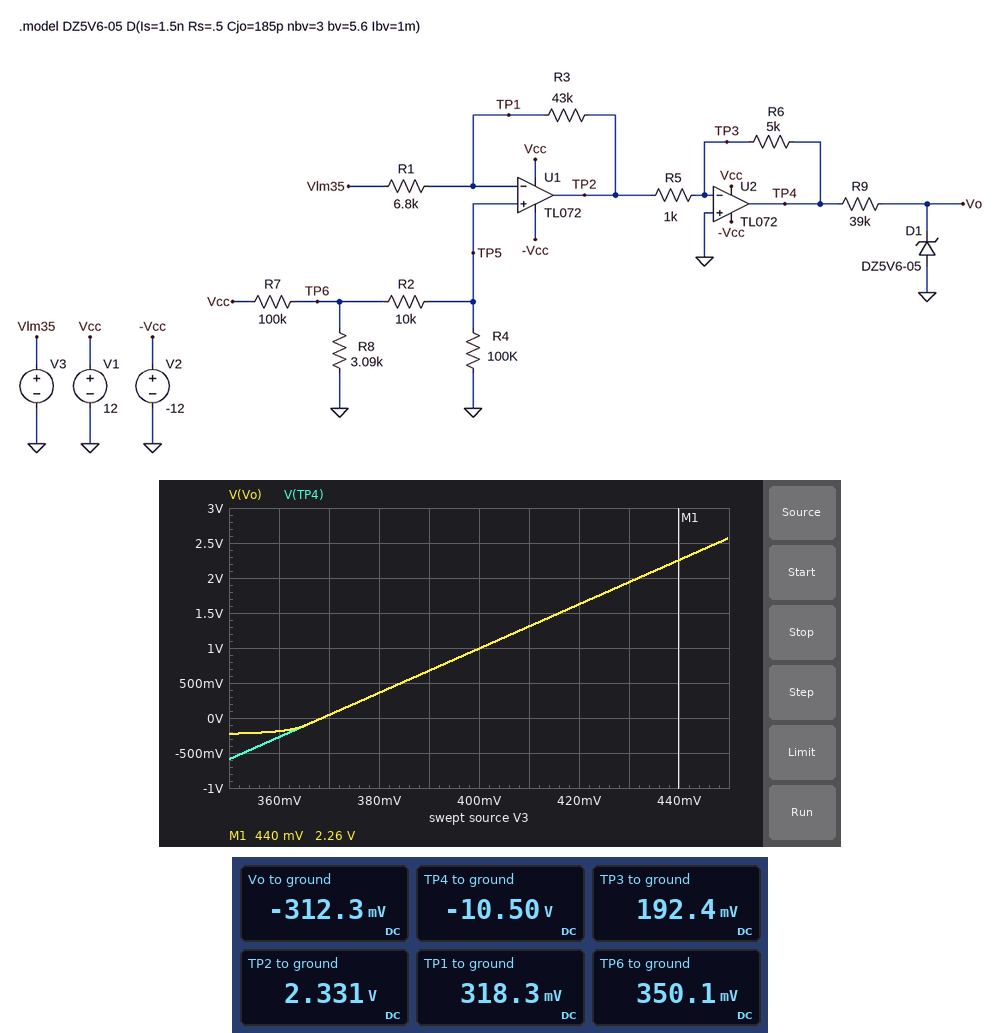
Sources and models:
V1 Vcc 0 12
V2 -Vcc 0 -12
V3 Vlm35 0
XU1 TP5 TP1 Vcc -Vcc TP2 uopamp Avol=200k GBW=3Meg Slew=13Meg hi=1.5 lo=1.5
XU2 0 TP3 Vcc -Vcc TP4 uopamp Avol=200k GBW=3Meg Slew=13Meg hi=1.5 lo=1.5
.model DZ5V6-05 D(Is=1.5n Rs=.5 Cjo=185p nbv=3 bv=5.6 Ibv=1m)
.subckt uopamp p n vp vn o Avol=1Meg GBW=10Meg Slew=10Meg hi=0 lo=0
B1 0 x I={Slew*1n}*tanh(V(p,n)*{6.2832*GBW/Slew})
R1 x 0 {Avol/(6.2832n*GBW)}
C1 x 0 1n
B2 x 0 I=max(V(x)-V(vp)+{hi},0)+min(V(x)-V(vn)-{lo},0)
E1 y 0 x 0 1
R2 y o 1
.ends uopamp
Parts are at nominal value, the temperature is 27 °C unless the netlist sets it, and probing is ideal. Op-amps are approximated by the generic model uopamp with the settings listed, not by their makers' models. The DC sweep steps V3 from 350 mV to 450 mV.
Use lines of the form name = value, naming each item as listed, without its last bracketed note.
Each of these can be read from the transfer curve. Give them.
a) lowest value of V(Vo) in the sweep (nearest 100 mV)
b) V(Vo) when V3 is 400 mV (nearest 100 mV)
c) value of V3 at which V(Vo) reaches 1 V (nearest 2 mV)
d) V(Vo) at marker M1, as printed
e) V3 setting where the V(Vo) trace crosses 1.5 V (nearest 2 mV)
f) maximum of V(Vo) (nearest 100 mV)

lowest value of V(Vo) in the sweep = -200 mV
V(Vo) when V3 is 400 mV = 1.0 V
value of V3 at which V(Vo) reaches 1 V = 400 mV
V(Vo) at marker M1, as printed = 2.26 V
V3 setting where the V(Vo) trace crosses 1.5 V = 416 mV
maximum of V(Vo) = 2.6 V
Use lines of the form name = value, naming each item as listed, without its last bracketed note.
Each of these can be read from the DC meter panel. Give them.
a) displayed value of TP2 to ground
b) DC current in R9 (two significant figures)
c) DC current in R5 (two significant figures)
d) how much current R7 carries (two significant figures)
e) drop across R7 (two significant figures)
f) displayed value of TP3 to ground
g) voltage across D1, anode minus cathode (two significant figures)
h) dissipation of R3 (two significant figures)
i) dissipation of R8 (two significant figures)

displayed value of TP2 to ground = 2.331 V
DC current in R9 = 260 µA
DC current in R5 = 2.1 mA
how much current R7 carries = 120 µA
drop across R7 = 12 V
displayed value of TP3 to ground = 192.4 mV
voltage across D1, anode minus cathode = 310 mV
dissipation of R3 = 94 µW
dissipation of R8 = 40 µW
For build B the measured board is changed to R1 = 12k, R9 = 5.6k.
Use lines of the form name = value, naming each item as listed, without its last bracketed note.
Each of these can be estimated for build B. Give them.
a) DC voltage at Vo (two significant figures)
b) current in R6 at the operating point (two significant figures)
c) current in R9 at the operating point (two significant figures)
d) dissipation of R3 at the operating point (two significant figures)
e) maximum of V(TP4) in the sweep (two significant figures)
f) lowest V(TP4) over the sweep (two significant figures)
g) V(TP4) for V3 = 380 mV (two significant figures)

DC voltage at Vo = -350 mV
current in R6 at the operating point = 1.5 mA
current in R9 at the operating point = 1.2 mA
dissipation of R3 at the operating point = 30 µW
maximum of V(TP4) in the sweep = 770 mV
lowest V(TP4) over the sweep = -1.0 V
V(TP4) for V3 = 380 mV = -490 mV
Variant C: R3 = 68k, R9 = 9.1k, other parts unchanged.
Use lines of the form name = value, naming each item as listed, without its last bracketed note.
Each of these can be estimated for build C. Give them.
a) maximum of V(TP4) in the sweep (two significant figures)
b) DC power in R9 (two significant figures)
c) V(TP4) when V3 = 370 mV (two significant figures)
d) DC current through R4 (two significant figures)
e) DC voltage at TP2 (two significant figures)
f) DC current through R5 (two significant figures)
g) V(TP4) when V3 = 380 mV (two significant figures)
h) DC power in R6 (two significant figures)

maximum of V(TP4) in the sweep = 5.0 V
DC power in R9 = 11 mW
V(TP4) when V3 = 370 mV = 990 mV
DC current through R4 = 3.2 µA
DC voltage at TP2 = 3.5 V
DC current through R5 = 2.3 mA
V(TP4) when V3 = 380 mV = 1.5 V
DC power in R6 = 27 mW
